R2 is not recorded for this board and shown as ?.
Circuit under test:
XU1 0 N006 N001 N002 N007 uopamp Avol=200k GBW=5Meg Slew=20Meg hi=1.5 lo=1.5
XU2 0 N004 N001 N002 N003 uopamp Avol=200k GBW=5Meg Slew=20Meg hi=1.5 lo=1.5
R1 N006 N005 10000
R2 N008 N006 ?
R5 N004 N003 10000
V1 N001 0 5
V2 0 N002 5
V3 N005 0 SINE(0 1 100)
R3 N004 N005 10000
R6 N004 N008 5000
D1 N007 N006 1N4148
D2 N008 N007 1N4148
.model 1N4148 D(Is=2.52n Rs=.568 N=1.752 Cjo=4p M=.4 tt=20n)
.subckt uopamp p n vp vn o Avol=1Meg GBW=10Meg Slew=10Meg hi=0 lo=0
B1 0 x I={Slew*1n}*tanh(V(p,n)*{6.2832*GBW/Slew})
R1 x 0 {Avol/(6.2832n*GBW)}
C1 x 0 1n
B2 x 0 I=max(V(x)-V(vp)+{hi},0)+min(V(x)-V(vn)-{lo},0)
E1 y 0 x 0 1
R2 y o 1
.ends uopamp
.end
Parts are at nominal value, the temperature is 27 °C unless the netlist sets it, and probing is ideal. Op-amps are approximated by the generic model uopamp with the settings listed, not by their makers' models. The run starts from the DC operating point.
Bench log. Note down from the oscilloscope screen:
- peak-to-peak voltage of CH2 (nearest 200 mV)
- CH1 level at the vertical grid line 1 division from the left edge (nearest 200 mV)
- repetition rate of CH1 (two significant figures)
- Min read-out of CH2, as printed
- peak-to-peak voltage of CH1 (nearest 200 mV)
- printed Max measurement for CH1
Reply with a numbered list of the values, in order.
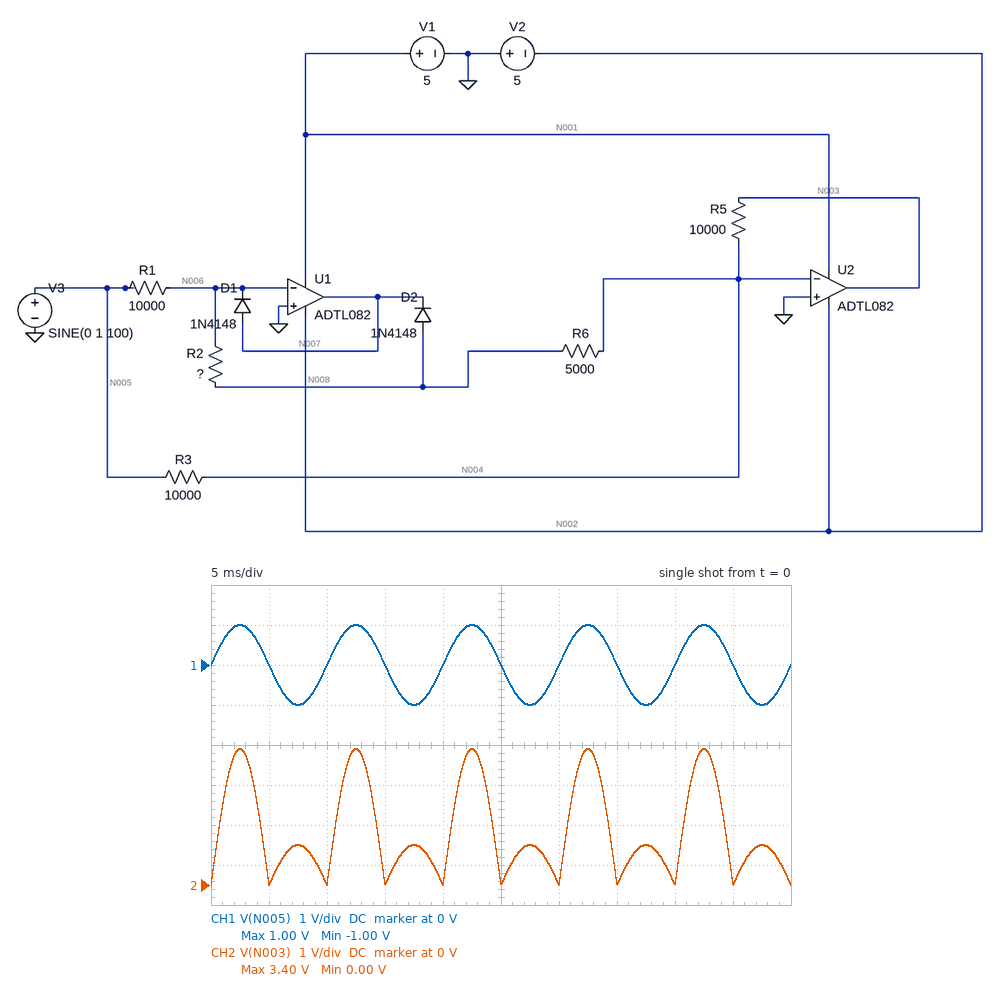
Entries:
1. 3.4 V
2. 0 V
3. 100 Hz
4. 0.00 V
5. 2.0 V
6. 1.00 V
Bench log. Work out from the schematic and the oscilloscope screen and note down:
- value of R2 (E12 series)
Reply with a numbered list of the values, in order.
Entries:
1. 22 kΩ
